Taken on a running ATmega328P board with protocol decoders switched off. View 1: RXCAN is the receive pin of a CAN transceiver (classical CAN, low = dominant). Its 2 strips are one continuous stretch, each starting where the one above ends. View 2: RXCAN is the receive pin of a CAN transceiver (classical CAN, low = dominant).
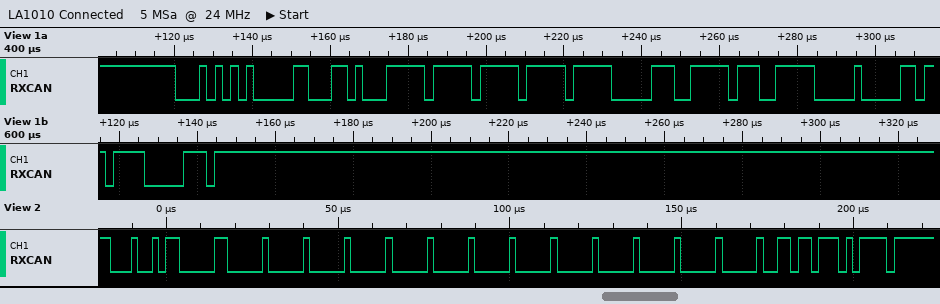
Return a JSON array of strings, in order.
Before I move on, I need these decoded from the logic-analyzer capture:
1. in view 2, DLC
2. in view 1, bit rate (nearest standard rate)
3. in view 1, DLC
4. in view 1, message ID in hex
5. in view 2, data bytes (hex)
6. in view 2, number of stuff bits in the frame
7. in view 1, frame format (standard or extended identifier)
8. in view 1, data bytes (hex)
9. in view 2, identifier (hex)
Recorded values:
["8", "500 kbit/s", "8", "0x154", "00 00 00 00 00 00 00 00", "14", "standard", "D1 FF FF FF 0C FF 3E 00", "0x12C"]
